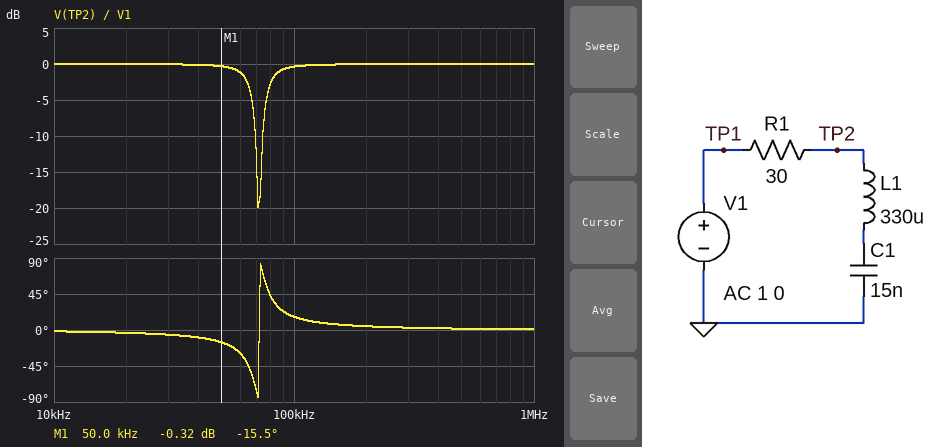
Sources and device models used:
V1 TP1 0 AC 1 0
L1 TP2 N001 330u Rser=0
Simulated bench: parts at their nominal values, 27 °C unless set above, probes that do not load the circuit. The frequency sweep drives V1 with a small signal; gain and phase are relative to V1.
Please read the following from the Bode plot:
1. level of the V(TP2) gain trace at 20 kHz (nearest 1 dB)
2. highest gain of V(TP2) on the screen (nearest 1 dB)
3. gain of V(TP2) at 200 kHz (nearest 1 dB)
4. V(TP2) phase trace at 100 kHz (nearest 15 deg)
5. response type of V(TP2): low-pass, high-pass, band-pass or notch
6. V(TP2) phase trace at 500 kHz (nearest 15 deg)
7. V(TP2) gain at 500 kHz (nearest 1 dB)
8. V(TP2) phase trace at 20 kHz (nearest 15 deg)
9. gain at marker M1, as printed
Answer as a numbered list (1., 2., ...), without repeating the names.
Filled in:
1. 0 dB
2. 0 dB
3. 0 dB
4. 15 deg
5. notch
6. 0 deg
7. 0 dB
8. 0 deg
9. -0.32 dB
